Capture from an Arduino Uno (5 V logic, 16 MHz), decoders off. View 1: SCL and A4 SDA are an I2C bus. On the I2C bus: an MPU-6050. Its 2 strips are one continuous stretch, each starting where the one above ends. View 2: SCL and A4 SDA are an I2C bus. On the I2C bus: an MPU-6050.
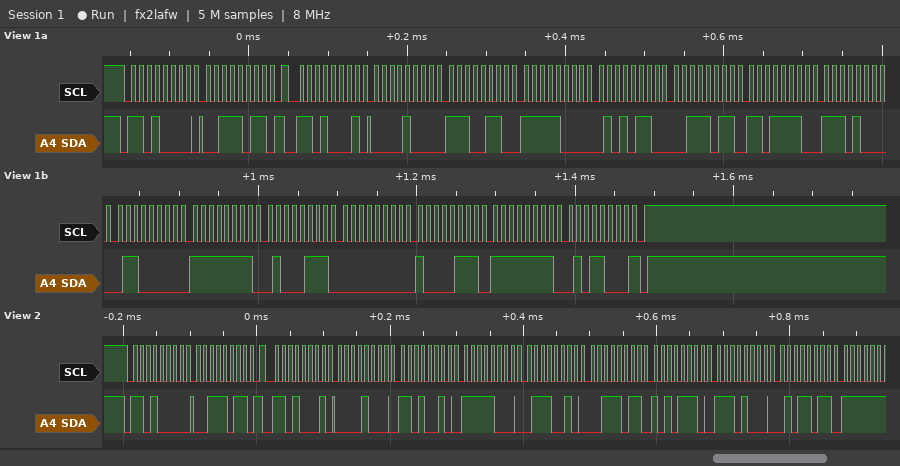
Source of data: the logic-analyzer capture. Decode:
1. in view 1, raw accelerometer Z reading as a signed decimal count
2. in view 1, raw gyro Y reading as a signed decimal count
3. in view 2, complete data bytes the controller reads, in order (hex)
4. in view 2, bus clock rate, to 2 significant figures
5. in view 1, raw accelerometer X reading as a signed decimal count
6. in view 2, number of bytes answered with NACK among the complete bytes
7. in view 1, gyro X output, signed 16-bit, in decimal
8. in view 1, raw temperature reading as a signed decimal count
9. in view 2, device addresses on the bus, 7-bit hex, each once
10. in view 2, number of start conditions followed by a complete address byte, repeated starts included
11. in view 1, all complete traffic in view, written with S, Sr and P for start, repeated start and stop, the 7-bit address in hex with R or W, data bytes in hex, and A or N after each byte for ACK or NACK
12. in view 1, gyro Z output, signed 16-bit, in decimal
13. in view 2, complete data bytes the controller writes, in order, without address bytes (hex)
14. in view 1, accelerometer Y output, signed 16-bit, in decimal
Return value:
15326
135
08 D2 F8 72 3B AE E8 5B
100 kHz
2278
0
-185
-6048
0x68
2
S 68W A 3B A Sr 68R A 08 A E6 A F8 A 56 A 3B A DE A E8 A 60 A FF A 47 A 00 A 87 A FF A 58 N P
-168
3B
-1962
